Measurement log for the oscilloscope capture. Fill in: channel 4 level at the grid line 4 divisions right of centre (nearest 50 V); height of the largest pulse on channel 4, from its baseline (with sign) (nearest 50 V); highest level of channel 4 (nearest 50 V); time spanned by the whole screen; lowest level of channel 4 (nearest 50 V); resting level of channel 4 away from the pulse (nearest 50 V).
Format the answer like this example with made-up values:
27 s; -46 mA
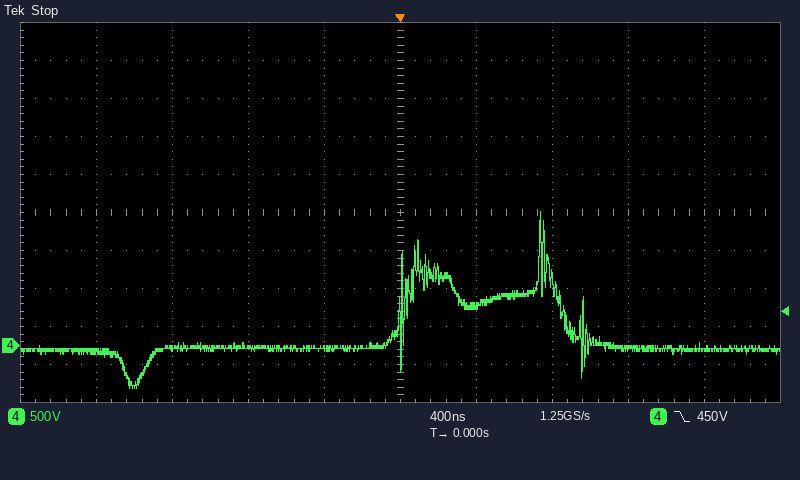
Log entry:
-50 V; +1.80 kV; 1.75 kV; 4 µs; -550 V; -50 V
